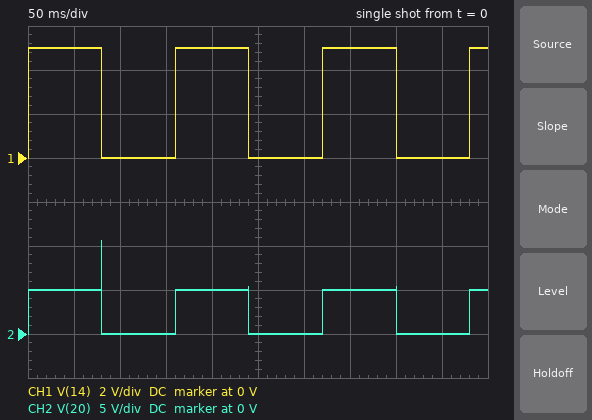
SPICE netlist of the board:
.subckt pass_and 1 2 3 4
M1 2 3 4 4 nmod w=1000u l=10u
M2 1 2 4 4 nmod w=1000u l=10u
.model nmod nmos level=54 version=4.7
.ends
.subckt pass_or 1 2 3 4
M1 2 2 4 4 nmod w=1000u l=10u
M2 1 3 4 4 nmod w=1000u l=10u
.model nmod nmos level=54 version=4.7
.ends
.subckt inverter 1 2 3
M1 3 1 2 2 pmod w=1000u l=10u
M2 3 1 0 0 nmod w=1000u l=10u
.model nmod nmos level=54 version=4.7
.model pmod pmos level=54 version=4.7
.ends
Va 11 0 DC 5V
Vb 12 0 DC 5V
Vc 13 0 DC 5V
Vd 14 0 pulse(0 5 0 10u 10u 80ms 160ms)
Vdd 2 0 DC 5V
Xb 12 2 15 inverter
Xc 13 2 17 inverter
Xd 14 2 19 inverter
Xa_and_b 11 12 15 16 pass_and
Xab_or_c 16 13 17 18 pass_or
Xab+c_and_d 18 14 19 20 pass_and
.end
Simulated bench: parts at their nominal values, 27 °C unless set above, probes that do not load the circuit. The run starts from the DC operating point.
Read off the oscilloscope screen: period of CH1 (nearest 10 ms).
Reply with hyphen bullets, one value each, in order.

- 160 ms
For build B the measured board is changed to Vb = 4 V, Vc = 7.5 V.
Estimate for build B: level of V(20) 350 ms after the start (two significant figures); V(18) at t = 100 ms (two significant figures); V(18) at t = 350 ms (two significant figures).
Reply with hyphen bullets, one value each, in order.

- 5.2 V
- 7.4 V
- 7.5 V
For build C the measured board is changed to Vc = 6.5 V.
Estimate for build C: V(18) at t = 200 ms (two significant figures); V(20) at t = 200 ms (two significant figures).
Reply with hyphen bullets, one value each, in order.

- 6.5 V
- 5.2 V
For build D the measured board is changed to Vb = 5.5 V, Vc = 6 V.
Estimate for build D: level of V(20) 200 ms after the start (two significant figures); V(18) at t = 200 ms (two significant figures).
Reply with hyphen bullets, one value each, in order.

- 5.2 V
- 6.0 V
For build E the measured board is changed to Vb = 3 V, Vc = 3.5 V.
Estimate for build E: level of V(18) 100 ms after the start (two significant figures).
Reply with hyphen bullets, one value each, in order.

- 3.5 V
